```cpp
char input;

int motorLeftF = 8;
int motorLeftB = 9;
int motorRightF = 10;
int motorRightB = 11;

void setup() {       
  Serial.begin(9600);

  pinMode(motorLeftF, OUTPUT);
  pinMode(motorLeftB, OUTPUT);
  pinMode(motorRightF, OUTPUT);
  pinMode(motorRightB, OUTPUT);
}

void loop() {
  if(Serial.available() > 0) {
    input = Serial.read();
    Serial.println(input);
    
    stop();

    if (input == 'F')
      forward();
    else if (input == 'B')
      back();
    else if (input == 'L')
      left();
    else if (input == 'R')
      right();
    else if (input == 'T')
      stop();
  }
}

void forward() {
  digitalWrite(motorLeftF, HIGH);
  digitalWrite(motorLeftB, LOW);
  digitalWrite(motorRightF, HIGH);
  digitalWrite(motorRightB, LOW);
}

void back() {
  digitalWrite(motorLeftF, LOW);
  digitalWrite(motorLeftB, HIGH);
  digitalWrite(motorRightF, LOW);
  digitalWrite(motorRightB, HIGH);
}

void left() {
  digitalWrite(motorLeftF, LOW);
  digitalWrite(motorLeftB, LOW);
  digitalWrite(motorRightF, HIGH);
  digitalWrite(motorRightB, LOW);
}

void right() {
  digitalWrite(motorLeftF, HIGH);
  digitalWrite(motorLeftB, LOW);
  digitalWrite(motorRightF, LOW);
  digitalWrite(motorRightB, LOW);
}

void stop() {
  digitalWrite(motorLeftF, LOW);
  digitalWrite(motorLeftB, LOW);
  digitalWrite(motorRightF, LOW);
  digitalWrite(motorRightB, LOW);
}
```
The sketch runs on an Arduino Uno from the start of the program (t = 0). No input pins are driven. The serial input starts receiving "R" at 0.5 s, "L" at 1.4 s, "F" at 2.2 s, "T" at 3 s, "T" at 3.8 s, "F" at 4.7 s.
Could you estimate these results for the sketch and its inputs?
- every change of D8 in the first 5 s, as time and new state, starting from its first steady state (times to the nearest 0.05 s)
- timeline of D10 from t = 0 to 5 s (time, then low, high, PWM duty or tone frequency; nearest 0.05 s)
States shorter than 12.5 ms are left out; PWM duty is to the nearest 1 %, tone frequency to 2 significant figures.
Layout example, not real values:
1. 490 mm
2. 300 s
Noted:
1. 0 s low; 0.5 s high; 1.4 s low; 2.2 s high; 3 s low; 4.7 s high
2. 0 s low; 1.4 s high; 3 s low; 4.7 s high
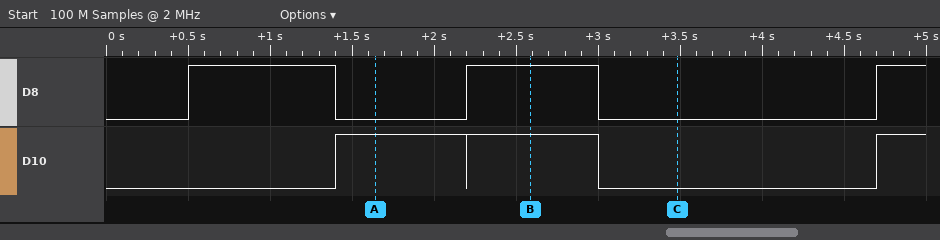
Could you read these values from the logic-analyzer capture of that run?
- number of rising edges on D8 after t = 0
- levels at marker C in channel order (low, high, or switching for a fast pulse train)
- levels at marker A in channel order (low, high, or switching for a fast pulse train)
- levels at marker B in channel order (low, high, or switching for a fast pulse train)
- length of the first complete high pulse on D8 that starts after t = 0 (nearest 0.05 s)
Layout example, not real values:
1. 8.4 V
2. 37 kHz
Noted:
1. 3
2. D8 low, D10 low
3. D8 low, D10 high
4. D8 high, D10 high
5. 0.90 s
